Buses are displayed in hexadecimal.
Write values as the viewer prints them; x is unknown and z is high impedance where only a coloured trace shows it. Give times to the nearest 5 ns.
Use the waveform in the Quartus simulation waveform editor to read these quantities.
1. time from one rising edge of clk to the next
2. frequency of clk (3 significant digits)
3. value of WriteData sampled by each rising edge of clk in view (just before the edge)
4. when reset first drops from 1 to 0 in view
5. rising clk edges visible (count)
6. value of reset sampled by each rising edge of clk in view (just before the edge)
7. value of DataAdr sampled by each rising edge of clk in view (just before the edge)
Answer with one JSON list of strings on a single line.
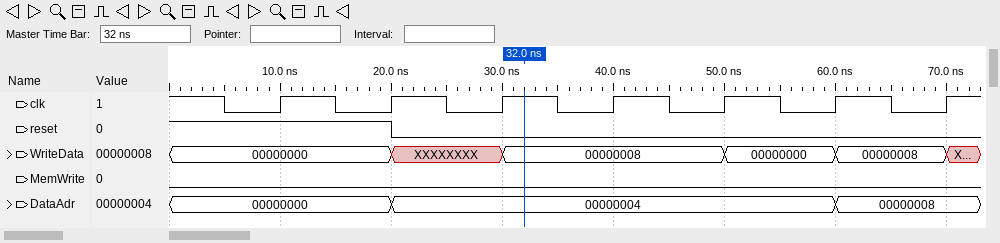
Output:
["10 ns", "100 MHz", "00000000, 00000000, XXXXXXXX, 00000008, 00000008, 00000000, 00000008", "20 ns", "7", "1 1 0 0 0 0 0", "00000000, 00000000, 00000004, 00000004, 00000004, 00000004, 00000008"]
